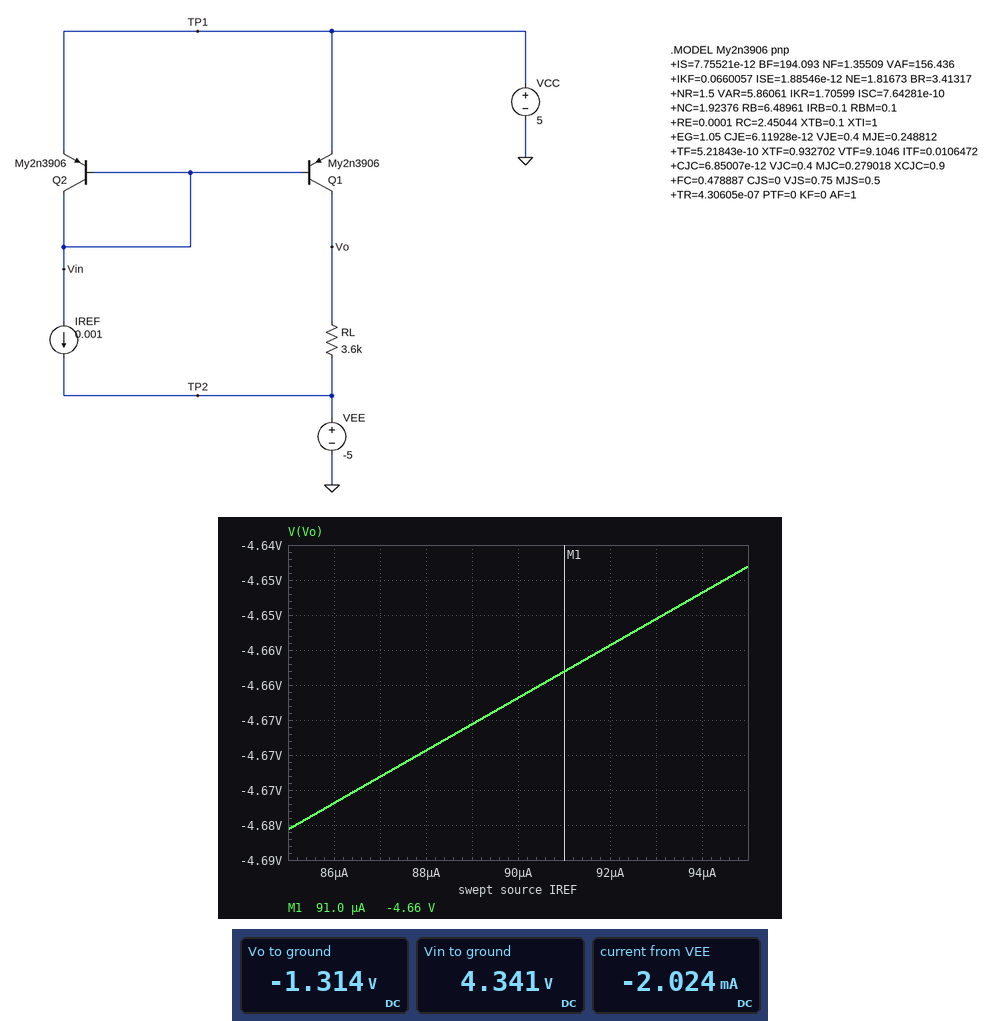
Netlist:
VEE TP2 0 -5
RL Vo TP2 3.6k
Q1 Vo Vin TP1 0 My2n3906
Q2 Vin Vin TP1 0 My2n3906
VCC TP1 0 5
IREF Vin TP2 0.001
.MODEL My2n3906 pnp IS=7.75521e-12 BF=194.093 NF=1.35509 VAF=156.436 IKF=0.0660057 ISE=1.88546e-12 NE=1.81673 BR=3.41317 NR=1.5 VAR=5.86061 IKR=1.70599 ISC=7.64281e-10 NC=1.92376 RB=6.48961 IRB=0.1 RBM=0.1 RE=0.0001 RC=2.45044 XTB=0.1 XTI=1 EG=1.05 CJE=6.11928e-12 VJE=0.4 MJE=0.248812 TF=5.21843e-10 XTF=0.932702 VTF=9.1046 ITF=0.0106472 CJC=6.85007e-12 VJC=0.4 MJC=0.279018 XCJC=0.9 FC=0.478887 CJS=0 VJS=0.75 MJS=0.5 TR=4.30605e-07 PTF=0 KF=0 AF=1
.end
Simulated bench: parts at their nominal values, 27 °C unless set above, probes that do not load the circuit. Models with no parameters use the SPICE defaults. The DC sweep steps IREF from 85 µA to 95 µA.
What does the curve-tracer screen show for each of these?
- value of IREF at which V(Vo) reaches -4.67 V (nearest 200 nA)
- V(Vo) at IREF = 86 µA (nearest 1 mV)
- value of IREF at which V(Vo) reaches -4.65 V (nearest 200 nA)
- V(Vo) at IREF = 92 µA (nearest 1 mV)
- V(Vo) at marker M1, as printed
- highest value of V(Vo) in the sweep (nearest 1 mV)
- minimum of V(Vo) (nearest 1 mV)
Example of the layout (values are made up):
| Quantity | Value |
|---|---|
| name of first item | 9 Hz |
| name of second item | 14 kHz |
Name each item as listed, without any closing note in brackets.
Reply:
| Quantity | Value |
|---|---|
| value of IREF at which V(Vo) reaches -4.67 V | 87.8 µA |
| V(Vo) at IREF = 86 µA | -4.677 V |
| value of IREF at which V(Vo) reaches -4.65 V | 93.2 µA |
| V(Vo) at IREF = 92 µA | -4.654 V |
| V(Vo) at marker M1, as printed | -4.66 V |
| highest value of V(Vo) in the sweep | -4.643 V |
| minimum of V(Vo) | -4.681 V |
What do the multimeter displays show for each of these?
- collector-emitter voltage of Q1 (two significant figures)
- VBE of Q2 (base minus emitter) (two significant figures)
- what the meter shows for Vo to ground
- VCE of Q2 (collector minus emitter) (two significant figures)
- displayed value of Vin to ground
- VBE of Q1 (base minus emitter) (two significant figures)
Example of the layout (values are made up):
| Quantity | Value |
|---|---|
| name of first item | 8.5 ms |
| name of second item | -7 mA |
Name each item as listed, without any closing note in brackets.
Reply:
| Quantity | Value |
|---|---|
| collector-emitter voltage of Q1 | -6.3 V |
| VBE of Q2 (base minus emitter) | -660 mV |
| what the meter shows for Vo to ground | -1.314 V |
| VCE of Q2 (collector minus emitter) | -660 mV |
| displayed value of Vin to ground | 4.341 V |
| VBE of Q1 (base minus emitter) | -660 mV |
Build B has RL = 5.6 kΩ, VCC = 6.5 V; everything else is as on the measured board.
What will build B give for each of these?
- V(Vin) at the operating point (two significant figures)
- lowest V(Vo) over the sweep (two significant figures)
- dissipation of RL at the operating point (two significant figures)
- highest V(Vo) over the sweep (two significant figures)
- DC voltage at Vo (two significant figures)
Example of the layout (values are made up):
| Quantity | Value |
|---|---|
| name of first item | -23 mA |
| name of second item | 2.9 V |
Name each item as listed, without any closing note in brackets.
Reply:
| Quantity | Value |
|---|---|
| V(Vin) at the operating point | 5.8 V |
| lowest V(Vo) over the sweep | -4.5 V |
| dissipation of RL at the operating point | 5.8 mW |
| highest V(Vo) over the sweep | -4.4 V |
| DC voltage at Vo | 710 mV |
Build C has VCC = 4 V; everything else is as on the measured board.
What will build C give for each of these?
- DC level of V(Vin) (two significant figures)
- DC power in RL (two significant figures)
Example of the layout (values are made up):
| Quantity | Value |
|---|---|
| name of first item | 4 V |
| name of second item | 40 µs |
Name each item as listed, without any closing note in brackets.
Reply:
| Quantity | Value |
|---|---|
| DC level of V(Vin) | 3.3 V |
| DC power in RL | 3.7 mW |
